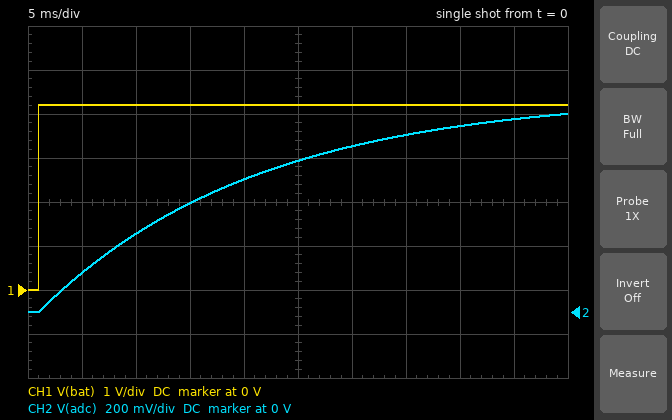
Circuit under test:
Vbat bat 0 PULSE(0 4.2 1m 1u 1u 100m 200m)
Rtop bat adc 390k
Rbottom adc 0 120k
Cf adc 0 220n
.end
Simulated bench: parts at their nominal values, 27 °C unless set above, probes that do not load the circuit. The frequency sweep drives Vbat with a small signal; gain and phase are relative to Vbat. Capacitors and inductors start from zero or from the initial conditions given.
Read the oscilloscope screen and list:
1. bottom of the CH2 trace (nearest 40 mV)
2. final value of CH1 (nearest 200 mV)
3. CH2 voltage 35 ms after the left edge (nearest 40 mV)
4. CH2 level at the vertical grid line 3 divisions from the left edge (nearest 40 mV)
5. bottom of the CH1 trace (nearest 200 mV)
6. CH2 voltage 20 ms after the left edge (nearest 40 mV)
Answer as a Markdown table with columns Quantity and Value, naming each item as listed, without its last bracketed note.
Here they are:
| Quantity | Value |
|---|---|
| bottom of the CH2 trace | 0 V |
| final value of CH1 | 4.2 V |
| CH2 voltage 35 ms after the left edge | 800 mV |
| CH2 level at the vertical grid line 3 divisions from the left edge | 480 mV |
| bottom of the CH1 trace | 0 V |
| CH2 voltage 20 ms after the left edge | 600 mV |
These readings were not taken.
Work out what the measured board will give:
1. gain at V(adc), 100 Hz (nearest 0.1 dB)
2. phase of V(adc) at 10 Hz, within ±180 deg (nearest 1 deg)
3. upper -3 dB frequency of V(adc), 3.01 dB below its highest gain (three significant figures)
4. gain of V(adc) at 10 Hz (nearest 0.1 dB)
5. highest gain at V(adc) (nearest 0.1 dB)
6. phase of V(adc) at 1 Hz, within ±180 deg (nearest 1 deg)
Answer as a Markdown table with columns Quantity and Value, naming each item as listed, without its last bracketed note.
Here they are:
| Quantity | Value |
|---|---|
| gain at V(adc), 100 Hz | -34.7 dB |
| phase of V(adc) at 10 Hz, within ±180 deg | -52 deg |
| upper -3 dB frequency of V(adc), 3.01 dB below its highest gain | 7.88 Hz |
| gain of V(adc) at 10 Hz | -16.7 dB |
| highest gain at V(adc) | -12.6 dB |
| phase of V(adc) at 1 Hz, within ±180 deg | -7 deg |
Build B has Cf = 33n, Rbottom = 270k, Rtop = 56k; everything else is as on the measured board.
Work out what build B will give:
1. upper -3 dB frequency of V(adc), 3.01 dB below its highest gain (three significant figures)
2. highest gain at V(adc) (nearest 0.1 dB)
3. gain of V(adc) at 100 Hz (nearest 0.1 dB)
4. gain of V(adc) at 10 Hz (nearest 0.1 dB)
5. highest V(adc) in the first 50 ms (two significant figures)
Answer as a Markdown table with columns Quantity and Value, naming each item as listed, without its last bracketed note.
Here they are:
| Quantity | Value |
|---|---|
| upper -3 dB frequency of V(adc), 3.01 dB below its highest gain | 104 Hz |
| highest gain at V(adc) | -1.6 dB |
| gain of V(adc) at 100 Hz | -4.5 dB |
| gain of V(adc) at 10 Hz | -1.7 dB |
| highest V(adc) in the first 50 ms | 3.5 V |
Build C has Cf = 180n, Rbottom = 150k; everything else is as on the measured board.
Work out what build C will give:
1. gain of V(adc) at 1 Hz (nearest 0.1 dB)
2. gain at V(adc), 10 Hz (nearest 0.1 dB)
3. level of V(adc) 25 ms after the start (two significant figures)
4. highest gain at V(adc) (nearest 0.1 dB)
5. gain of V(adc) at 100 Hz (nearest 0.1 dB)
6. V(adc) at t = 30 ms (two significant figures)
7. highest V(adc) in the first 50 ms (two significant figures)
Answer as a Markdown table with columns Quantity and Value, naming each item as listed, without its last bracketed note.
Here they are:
| Quantity | Value |
|---|---|
| gain of V(adc) at 1 Hz | -11.2 dB |
| gain at V(adc), 10 Hz | -15.1 dB |
| level of V(adc) 25 ms after the start | 830 mV |
| highest gain at V(adc) | -11.1 dB |
| gain of V(adc) at 100 Hz | -32.9 dB |
| V(adc) at t = 30 ms | 900 mV |
| highest V(adc) in the first 50 ms | 1.1 V |
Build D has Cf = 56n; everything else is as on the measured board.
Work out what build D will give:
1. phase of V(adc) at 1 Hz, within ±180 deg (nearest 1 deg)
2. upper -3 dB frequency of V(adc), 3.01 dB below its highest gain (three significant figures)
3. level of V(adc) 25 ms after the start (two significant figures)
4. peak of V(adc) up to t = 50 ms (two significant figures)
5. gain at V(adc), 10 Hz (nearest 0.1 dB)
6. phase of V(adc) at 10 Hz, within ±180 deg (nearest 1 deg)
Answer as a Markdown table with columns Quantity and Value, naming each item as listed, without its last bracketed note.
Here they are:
| Quantity | Value |
|---|---|
| phase of V(adc) at 1 Hz, within ±180 deg | -2 deg |
| upper -3 dB frequency of V(adc), 3.01 dB below its highest gain | 31.0 Hz |
| level of V(adc) 25 ms after the start | 980 mV |
| peak of V(adc) up to t = 50 ms | 990 mV |
| gain at V(adc), 10 Hz | -13.0 dB |
| phase of V(adc) at 10 Hz, within ±180 deg | -18 deg |
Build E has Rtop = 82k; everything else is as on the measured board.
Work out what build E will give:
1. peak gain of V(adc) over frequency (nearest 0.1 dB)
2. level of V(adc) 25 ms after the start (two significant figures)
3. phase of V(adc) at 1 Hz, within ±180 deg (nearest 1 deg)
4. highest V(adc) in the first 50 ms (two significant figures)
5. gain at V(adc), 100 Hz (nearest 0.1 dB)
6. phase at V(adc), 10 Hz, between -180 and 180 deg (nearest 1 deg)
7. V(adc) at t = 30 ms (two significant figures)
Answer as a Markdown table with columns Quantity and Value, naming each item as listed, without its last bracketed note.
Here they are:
| Quantity | Value |
|---|---|
| peak gain of V(adc) over frequency | -4.5 dB |
| level of V(adc) 25 ms after the start | 2.2 V |
| phase of V(adc) at 1 Hz, within ±180 deg | -4 deg |
| highest V(adc) in the first 50 ms | 2.5 V |
| gain at V(adc), 100 Hz | -21.2 dB |
| phase at V(adc), 10 Hz, between -180 and 180 deg | -34 deg |
| V(adc) at t = 30 ms | 2.3 V |
